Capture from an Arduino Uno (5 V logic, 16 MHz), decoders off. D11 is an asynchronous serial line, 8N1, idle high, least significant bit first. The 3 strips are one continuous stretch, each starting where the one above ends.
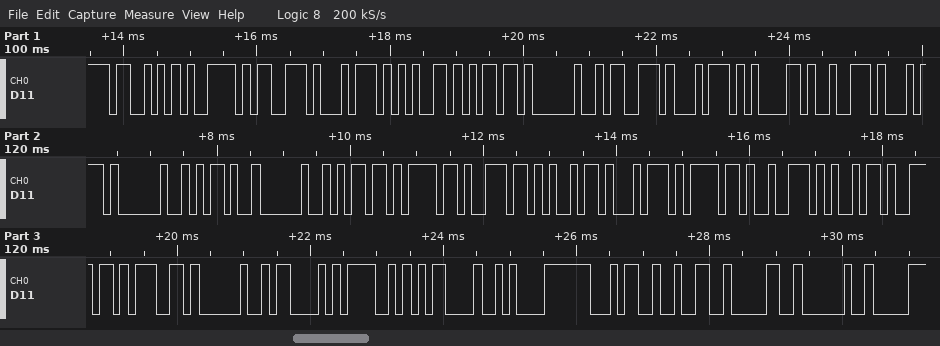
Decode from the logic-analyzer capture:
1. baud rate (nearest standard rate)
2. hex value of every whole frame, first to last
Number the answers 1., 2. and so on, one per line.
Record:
1. 9600 baud
2. 53 79 73 74 65 6D 20 73 74 61 72 74 20 2D 20 6D 6F 6E 69 74 6F 72 69 6E 67 20 43 4F 0D 0A 34 32 30 20
